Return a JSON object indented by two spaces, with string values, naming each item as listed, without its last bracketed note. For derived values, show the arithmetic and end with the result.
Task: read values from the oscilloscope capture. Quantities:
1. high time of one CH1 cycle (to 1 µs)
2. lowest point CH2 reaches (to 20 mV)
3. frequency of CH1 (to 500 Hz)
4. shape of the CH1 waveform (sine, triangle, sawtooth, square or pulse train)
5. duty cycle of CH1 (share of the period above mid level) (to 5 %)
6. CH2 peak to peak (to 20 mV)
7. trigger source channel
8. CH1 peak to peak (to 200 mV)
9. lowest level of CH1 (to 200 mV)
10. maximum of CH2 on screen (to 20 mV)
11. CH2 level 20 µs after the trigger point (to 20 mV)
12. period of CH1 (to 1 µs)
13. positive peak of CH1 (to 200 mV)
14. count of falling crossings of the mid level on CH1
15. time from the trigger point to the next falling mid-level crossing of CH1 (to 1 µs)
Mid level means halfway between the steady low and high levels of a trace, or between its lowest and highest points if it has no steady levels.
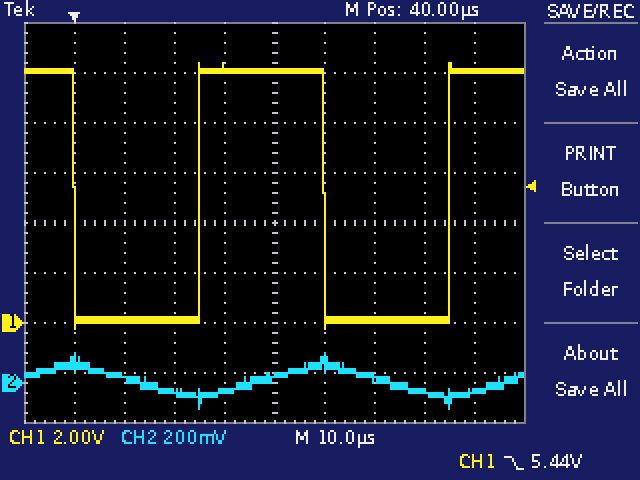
{
  "high time of one CH1 cycle": "25 µs",
  "lowest point CH2 reaches": "-100 mV",
  "frequency of CH1": "1 / 50 µs ≈ 20.0 kHz",
  "shape of the CH1 waveform": "square",
  "duty cycle of CH1 (share of the period above mid level)": "25 µs / 50 µs ≈ 50 %",
  "CH2 peak to peak": "120 mV − (-100 mV) = 220 mV",
  "trigger source channel": "CH1",
  "CH1 peak to peak": "10.4 V − (-200 mV) = 10.6 V",
  "lowest level of CH1": "-200 mV",
  "maximum of CH2 on screen": "120 mV",
  "CH2 level 20 µs after the trigger point": "-40 mV",
  "period of CH1": "50 µs",
  "positive peak of CH1": "10.4 V",
  "count of falling crossings of the mid level on CH1": "2",
  "time from the trigger point to the next falling mid-level crossing of CH1": "50 µs"
}
